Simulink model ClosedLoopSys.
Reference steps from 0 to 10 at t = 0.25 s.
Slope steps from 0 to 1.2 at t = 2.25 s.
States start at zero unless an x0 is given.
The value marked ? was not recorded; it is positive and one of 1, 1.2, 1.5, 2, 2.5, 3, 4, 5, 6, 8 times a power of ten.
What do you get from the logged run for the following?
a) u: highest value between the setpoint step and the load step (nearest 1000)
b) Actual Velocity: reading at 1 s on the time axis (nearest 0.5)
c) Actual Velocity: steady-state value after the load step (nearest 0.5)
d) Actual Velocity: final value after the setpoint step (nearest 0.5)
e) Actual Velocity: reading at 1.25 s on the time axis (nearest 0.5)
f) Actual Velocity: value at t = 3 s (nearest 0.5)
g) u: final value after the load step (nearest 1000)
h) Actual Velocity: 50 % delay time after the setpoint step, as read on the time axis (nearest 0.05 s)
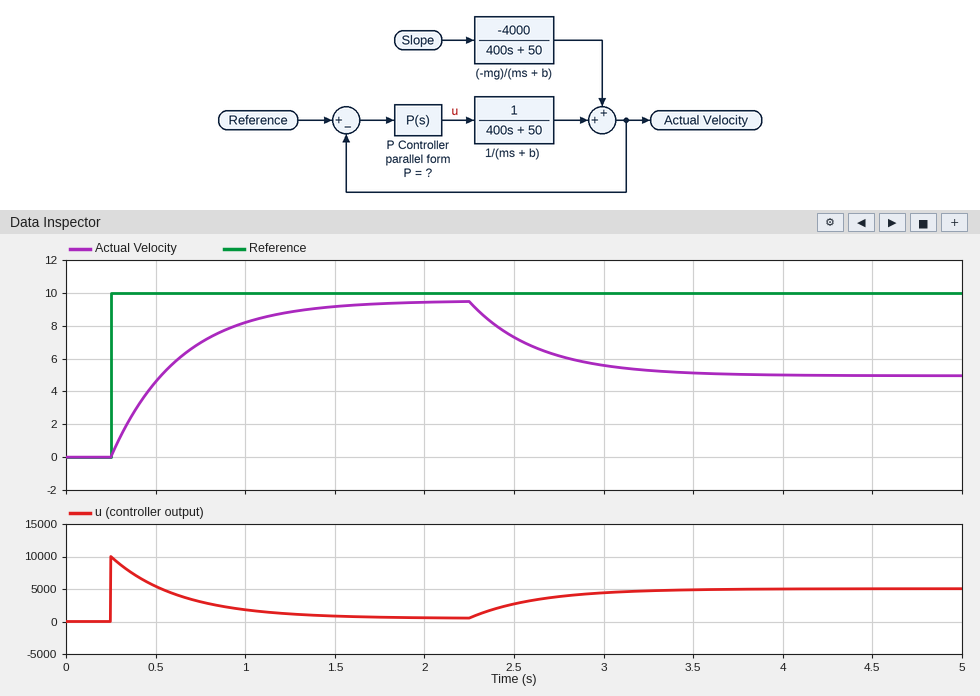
10000
8.0
5.0
9.5
9.0
5.5
5000
0.50 s
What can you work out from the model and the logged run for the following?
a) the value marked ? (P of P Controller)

1000
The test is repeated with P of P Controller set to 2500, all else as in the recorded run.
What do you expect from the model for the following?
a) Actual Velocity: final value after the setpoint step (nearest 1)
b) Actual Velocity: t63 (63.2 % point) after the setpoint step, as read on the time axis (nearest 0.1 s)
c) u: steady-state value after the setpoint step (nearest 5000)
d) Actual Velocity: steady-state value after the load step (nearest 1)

10
0.4 s
0
8
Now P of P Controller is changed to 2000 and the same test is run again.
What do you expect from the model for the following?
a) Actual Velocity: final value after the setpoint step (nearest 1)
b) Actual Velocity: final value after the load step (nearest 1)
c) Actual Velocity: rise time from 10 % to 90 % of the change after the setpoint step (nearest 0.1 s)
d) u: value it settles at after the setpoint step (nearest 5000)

10
7
0.4 s
0
